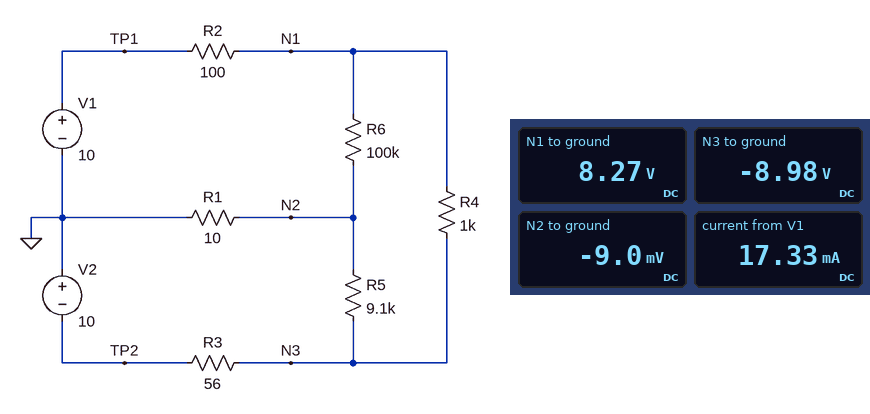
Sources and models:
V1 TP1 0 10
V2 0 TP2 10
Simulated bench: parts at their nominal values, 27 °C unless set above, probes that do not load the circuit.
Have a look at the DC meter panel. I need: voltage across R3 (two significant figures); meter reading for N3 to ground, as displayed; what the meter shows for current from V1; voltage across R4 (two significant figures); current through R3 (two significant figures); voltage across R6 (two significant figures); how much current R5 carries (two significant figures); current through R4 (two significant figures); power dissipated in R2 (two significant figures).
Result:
1.0 V
-8.98 V
17.33 mA
17 V
18 mA
8.3 V
990 µA
17 mA
30 mW
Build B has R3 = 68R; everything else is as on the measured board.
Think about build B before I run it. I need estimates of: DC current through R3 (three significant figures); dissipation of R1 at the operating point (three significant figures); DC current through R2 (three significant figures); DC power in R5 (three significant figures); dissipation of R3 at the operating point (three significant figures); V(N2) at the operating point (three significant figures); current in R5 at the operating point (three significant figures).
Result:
18.0 mA
7.75 µW
17.1 mA
8.44 mW
22.1 mW
-8.80 mV
963 µA
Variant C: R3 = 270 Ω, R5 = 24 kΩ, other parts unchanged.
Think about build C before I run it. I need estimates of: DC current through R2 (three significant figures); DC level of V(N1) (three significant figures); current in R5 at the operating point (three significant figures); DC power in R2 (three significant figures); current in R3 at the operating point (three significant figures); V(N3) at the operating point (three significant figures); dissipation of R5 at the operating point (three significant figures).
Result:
14.6 mA
8.54 V
250 µA
21.4 mW
14.8 mA
-6.01 V
1.50 mW
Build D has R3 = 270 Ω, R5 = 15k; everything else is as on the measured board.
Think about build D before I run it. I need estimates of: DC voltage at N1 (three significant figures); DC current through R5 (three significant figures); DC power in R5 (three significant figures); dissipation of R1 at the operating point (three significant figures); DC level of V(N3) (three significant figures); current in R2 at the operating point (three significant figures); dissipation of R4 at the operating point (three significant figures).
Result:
8.54 V
398 µA
2.38 mW
977 nW
-5.97 V
14.6 mA
211 mW
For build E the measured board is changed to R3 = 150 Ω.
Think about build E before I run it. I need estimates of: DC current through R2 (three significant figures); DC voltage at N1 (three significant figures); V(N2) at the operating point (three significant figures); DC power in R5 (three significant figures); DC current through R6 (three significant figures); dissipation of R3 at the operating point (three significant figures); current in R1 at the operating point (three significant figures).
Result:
16.0 mA
8.40 V
-7.38 mV
6.16 mW
84.1 µA
41.9 mW
738 µA
